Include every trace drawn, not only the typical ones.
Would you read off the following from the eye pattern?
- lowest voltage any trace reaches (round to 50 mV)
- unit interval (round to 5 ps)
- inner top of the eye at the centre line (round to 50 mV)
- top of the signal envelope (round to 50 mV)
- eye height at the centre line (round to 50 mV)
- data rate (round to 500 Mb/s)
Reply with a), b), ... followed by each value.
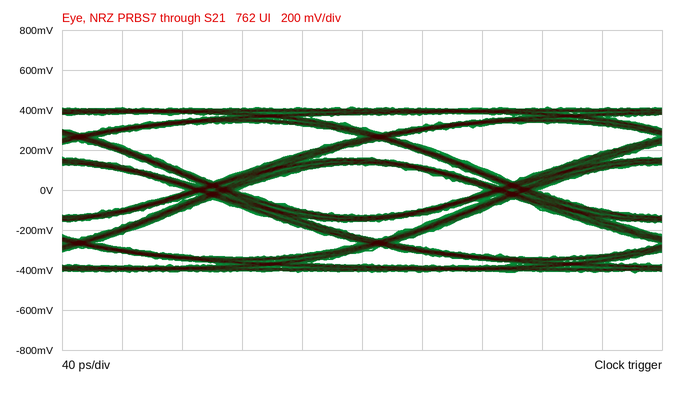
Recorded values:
a) -400 mV
b) 200 ps
c) 150 mV
d) 400 mV
e) 250 mV
f) 5.0 Gb/s
